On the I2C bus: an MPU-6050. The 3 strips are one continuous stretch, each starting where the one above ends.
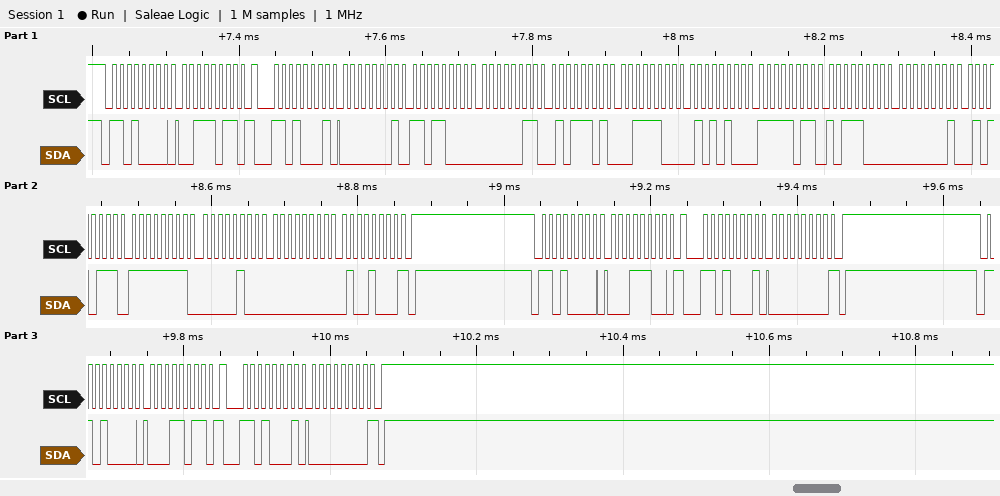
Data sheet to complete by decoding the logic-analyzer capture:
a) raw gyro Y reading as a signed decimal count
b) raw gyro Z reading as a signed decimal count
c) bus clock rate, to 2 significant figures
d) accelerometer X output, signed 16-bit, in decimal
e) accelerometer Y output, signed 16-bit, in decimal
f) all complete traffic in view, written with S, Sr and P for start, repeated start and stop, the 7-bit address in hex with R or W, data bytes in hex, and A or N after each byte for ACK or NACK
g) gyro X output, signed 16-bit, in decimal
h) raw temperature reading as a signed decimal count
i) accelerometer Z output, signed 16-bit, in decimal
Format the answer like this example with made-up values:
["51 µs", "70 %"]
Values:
["-252", "72", "100 kHz", "472", "861", "S 68W A 3B A Sr 68R A 01 A D8 A 03 A 5D A 3C A 54 A FB A B8 A 01 A 57 A FF A 04 A 00 A 48 N P S 68W A 1C A Sr 68R A 00 N P S 68W A 1B A Sr 68R A 00 N P", "343", "-1096", "15444"]
